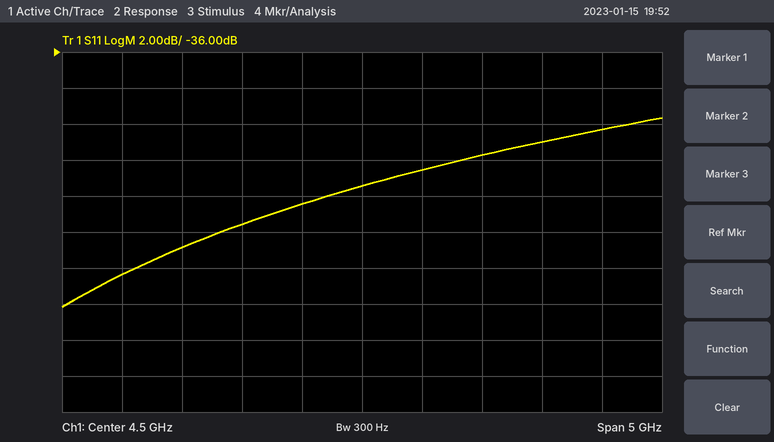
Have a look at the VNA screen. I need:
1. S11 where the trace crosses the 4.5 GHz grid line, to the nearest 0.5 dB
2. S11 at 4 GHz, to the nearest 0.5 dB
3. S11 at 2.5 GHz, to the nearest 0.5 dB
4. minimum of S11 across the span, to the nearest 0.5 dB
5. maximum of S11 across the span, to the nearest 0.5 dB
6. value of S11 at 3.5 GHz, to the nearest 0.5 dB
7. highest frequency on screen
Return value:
-43.5 dB
-44.5 dB
-48.5 dB
-50.0 dB
-39.5 dB
-45.5 dB
7 GHz
